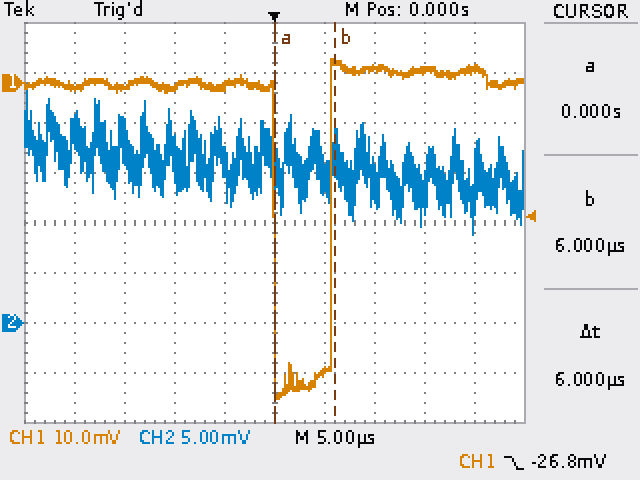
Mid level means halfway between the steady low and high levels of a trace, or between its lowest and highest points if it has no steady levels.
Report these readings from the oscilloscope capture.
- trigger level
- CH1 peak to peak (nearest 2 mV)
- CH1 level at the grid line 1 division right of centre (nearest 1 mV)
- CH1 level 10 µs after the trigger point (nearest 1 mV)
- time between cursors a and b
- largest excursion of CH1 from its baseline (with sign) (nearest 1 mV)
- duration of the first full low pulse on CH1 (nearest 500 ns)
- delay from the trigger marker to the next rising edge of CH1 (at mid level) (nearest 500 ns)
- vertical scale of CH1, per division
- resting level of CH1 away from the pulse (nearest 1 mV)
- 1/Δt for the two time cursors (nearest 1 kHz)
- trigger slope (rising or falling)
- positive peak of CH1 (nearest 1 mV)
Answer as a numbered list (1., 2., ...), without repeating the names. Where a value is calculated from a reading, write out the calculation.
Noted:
1. -26.8 mV
2. 68 mV
3. -58 mV
4. 3 mV
5. 6 µs
6. -63 mV
7. 5.5 µs
8. 5.5 µs
9. 10 mV
10. 0 mV
11. 1 / 6 µs ≈ 167 kHz
12. falling
13. 5 mV
